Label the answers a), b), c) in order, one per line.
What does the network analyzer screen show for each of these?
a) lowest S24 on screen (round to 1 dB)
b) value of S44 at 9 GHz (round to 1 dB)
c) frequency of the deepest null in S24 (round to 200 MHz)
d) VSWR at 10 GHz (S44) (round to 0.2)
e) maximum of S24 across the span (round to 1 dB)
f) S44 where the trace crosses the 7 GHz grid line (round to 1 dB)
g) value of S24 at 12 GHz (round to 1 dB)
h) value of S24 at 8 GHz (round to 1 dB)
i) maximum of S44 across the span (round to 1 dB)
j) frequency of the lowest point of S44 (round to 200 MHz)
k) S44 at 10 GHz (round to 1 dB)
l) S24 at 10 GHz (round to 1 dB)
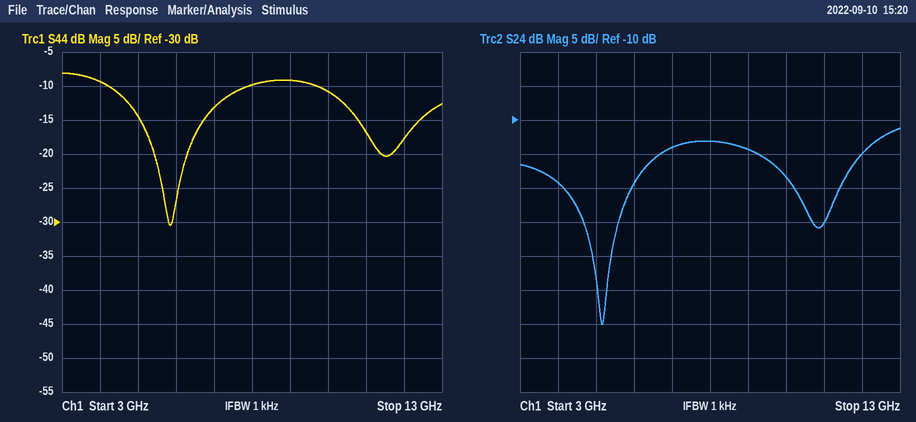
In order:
a) -40 dB
b) -9 dB
c) 5.2 GHz
d) 1.8
e) -11 dB
f) -13 dB
g) -15 dB
h) -13 dB
i) -8 dB
j) 5.8 GHz
k) -11 dB
l) -18 dB
